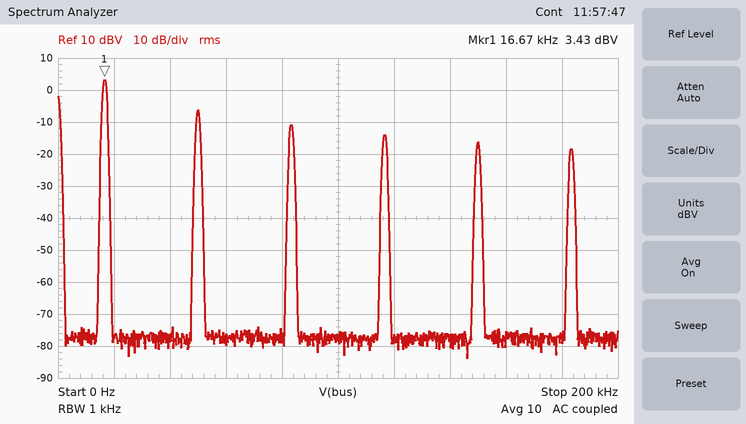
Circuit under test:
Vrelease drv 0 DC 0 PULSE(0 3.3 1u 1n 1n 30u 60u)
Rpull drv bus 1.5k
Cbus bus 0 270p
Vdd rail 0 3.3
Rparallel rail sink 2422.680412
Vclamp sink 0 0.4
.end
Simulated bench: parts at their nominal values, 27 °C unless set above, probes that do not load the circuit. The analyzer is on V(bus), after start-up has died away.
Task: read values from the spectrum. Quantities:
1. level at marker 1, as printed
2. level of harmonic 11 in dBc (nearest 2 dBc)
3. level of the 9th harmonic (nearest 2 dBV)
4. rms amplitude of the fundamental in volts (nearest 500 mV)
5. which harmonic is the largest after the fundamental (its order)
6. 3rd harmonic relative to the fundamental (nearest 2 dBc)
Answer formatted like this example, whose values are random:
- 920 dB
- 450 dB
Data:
- 3.43 dBV
- -22 dBc
- -16 dBV
- 1.5 V
- 3
- -10 dBc
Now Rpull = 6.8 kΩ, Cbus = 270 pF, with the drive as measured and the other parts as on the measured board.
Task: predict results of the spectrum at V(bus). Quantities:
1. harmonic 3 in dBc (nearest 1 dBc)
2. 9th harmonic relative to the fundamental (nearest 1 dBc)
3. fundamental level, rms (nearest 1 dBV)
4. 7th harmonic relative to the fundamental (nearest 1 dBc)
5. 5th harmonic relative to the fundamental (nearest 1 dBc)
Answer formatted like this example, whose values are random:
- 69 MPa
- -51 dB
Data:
- -11 dBc
- -25 dBc
- 3 dBV
- -21 dBc
- -17 dBc
